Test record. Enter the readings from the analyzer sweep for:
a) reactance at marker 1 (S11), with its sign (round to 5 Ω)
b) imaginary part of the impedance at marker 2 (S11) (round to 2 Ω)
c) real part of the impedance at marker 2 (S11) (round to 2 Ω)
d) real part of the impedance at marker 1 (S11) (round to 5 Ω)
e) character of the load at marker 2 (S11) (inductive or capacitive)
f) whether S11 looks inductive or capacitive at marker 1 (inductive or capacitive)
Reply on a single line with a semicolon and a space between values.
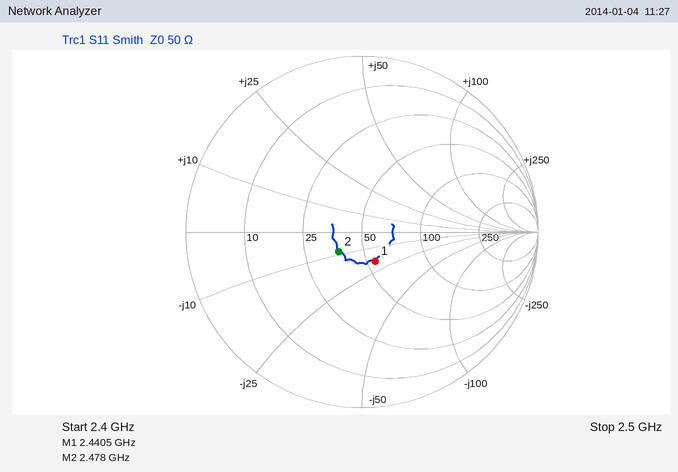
-20 Ω; -8 Ω; 38 Ω; 55 Ω; capacitive; capacitive
